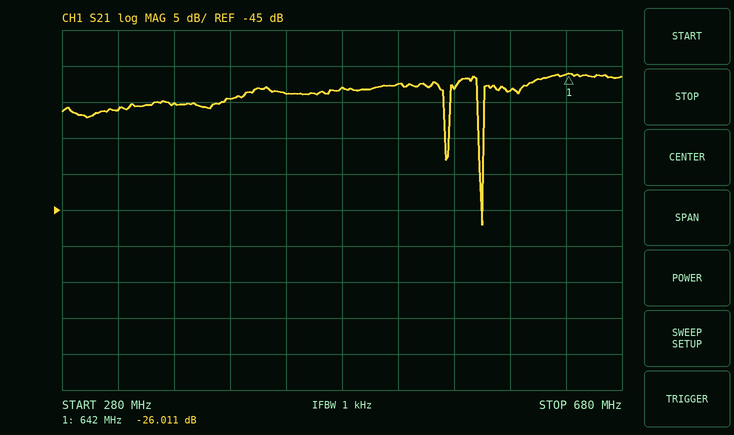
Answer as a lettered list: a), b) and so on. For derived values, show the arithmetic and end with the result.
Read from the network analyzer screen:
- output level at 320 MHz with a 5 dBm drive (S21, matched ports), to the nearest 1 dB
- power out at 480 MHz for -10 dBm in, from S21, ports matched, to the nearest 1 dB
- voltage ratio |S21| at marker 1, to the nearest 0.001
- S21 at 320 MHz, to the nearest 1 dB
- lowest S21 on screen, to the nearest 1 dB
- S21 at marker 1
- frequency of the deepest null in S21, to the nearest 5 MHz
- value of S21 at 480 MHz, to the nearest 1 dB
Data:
a) 5 dBm + (-31 dB) = -26 dBm
b) -10 dBm + (-28 dB) = -38 dBm
c) 10^(-26.011/20) ≈ 0.050
d) -31 dB
e) -47 dB
f) -26.011 dB
g) 580 MHz
h) -28 dB
